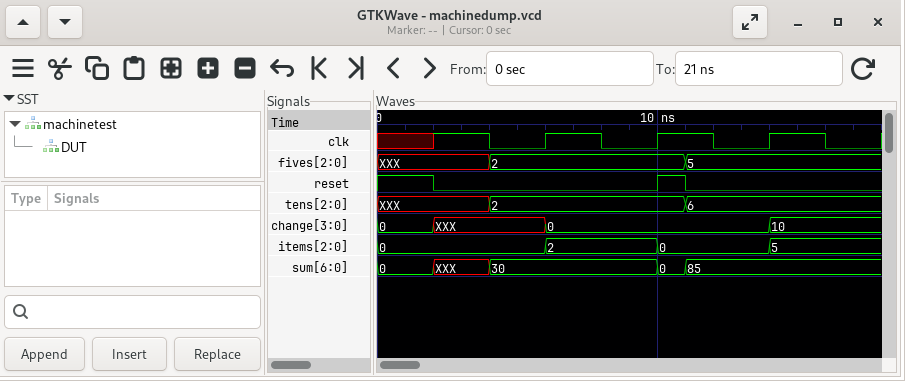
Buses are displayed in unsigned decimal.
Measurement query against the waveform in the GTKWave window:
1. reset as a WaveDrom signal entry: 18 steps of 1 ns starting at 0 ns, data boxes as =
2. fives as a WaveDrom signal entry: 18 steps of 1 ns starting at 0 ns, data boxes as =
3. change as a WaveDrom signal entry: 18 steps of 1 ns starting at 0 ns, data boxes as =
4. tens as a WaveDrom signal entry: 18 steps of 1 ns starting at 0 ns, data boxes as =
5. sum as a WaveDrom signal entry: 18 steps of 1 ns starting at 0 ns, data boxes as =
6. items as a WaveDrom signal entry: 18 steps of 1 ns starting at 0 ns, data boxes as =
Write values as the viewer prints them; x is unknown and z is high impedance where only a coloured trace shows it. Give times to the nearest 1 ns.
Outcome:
{name: 'reset', wave: '1.0.......10......'}
{name: 'fives', wave: 'x...=......=......', data: '2 5'}
{name: 'change', wave: '=.x...=.......=...', data: '0 0 10'}
{name: 'tens', wave: 'x...=......=......', data: '2 6'}
{name: 'sum', wave: '=.x.=.....==......', data: '0 30 0 85'}
{name: 'items', wave: '=.....=...=...=...', data: '0 2 0 5'}
